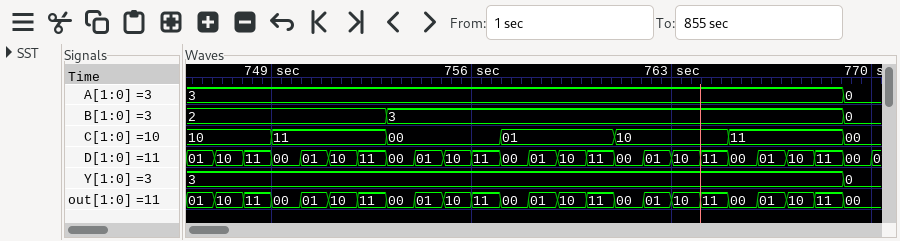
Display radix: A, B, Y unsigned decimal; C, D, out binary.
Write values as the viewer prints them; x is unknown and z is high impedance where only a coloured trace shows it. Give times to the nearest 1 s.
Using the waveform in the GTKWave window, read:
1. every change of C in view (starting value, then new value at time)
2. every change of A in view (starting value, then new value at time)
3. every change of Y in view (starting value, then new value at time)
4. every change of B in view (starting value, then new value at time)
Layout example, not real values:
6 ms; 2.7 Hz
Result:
10, 11 at 749 s, 00 at 753 s, 01 at 757 s, 10 at 761 s, 11 at 765 s, 00 at 769 s; 3, 0 at 769 s; 3, 0 at 769 s; 2, 3 at 753 s, 0 at 769 s
